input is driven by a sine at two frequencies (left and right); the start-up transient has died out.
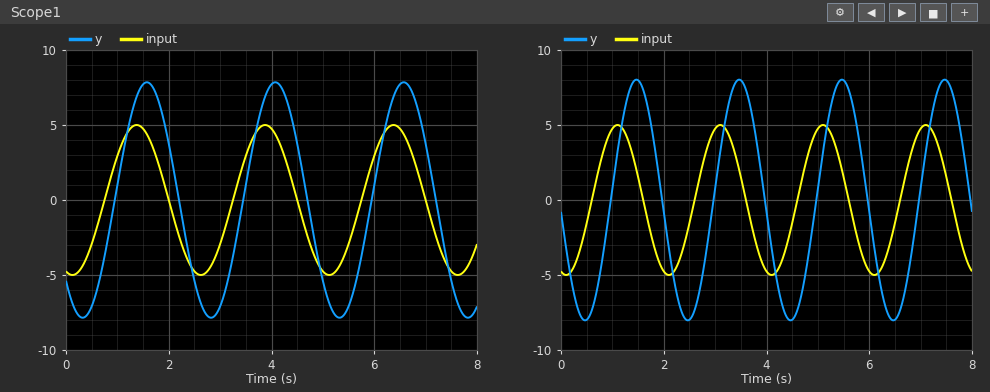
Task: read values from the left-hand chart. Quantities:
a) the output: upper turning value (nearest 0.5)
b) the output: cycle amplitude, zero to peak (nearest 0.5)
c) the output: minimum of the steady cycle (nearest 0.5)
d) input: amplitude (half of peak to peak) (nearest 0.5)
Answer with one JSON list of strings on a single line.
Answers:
["8.0", "8.0", "-8.0", "5.0"]
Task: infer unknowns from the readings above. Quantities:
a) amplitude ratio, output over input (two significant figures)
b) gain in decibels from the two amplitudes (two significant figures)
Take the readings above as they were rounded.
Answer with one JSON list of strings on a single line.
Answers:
["1.6", "4.1 dB"]
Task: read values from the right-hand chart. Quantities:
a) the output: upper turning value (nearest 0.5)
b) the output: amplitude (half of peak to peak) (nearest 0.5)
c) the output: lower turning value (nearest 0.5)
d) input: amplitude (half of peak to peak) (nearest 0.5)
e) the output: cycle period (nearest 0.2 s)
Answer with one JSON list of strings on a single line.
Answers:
["8.0", "8.0", "-8.0", "5.0", "2.0 s"]
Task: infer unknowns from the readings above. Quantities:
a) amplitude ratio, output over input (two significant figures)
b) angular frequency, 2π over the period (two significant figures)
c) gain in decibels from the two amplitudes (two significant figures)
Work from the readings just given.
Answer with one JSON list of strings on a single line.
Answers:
["1.6", "3.1 rad/s", "4.1 dB"]
